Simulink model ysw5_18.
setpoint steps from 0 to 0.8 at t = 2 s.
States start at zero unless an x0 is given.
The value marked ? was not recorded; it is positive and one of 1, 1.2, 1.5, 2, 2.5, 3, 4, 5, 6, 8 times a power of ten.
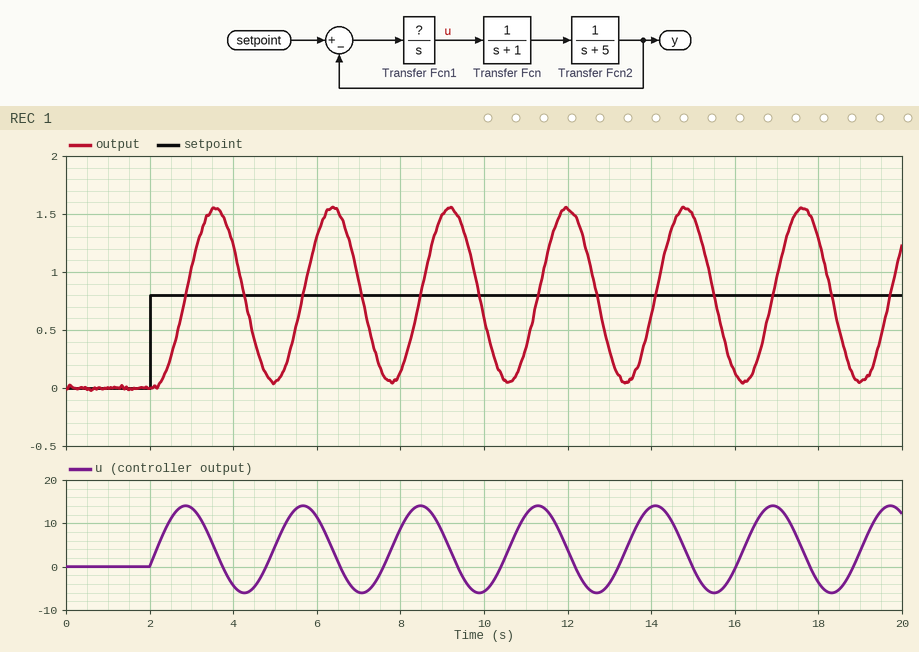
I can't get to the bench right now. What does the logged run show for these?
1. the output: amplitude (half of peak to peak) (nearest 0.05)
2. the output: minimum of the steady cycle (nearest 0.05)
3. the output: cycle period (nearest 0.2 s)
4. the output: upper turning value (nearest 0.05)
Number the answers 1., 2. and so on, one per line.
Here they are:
1. 0.75
2. 0.05
3. 2.8 s
4. 1.55
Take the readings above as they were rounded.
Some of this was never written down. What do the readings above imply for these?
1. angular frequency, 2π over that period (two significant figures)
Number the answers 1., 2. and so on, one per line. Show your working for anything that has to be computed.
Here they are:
1. 2π / 2.8 = 2.2 rad/s
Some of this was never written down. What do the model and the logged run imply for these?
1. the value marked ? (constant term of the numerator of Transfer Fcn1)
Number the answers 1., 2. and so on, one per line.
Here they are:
1. 30
